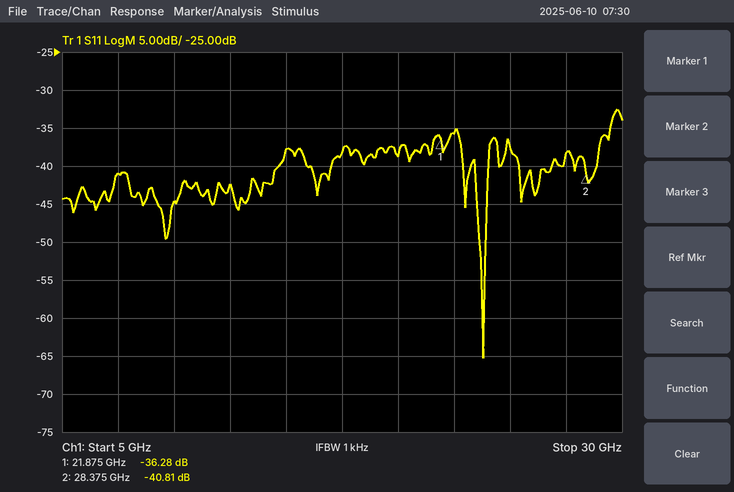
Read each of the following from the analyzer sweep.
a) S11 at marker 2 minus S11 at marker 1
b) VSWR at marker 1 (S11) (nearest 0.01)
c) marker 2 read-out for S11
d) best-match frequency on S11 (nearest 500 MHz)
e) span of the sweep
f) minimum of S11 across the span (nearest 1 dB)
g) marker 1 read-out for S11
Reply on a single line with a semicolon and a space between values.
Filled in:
-4.53 dB; 1.03; -40.81 dB; 24.0 GHz; 25 GHz; -65 dB; -36.28 dB
